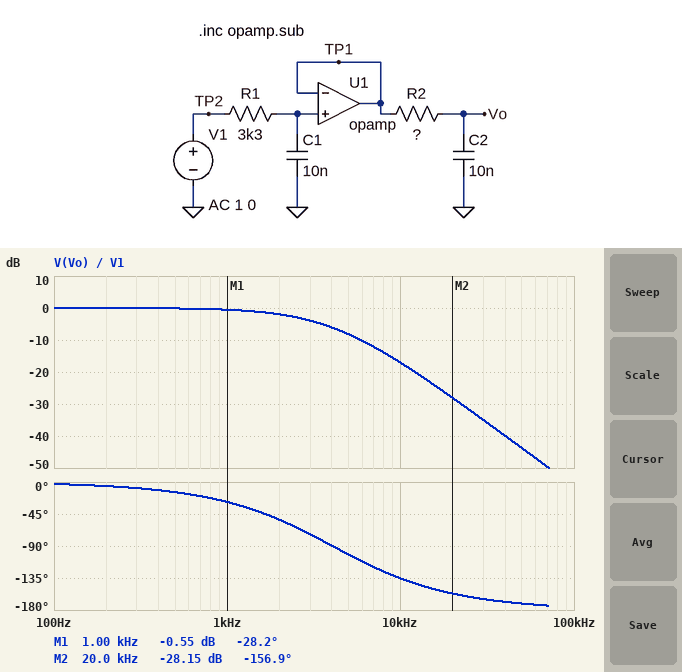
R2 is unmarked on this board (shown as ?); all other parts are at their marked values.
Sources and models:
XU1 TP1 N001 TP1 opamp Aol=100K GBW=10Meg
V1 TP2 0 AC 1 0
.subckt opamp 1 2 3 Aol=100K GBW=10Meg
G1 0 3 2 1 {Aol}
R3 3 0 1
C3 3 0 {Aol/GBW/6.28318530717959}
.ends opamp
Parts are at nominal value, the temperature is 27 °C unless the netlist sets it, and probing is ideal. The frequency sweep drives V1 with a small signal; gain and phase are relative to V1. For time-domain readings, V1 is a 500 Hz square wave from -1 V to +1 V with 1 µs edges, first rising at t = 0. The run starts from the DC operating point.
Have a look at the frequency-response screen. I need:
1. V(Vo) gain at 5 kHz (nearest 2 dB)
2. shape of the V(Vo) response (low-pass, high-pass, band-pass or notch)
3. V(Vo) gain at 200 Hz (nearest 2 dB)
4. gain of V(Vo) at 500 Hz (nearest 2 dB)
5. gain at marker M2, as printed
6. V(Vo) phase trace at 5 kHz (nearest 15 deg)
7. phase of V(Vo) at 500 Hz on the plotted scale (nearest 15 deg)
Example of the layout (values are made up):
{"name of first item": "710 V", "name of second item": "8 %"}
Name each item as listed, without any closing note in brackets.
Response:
{"V(Vo) gain at 5 kHz": "-8 dB", "shape of the V(Vo) response": "low-pass", "V(Vo) gain at 200 Hz": "0 dB", "gain of V(Vo) at 500 Hz": "0 dB", "gain at marker M2, as printed": "-28.15 dB", "V(Vo) phase trace at 5 kHz": "-105 deg", "phase of V(Vo) at 500 Hz on the plotted scale": "-15 deg"}
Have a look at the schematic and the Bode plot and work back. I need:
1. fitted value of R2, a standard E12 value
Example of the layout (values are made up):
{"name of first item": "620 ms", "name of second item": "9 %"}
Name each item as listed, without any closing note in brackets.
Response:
{"fitted value of R2, a standard E12 value": "4.7 kΩ"}
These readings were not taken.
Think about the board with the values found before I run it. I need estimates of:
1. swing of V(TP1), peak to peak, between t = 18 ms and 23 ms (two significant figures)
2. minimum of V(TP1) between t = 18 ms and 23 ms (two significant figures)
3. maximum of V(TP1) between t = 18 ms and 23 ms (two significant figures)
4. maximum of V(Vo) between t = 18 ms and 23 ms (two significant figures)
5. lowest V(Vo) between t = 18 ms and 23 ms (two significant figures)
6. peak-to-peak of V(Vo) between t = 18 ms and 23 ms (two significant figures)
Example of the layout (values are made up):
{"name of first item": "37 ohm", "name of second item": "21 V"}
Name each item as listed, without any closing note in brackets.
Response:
{"swing of V(TP1), peak to peak, between t = 18 ms and 23 ms": "2.0 V", "minimum of V(TP1) between t = 18 ms and 23 ms": "-1.0 V", "maximum of V(TP1) between t = 18 ms and 23 ms": "1.0 V", "maximum of V(Vo) between t = 18 ms and 23 ms": "1.0 V", "lowest V(Vo) between t = 18 ms and 23 ms": "-1.0 V", "peak-to-peak of V(Vo) between t = 18 ms and 23 ms": "2.0 V"}
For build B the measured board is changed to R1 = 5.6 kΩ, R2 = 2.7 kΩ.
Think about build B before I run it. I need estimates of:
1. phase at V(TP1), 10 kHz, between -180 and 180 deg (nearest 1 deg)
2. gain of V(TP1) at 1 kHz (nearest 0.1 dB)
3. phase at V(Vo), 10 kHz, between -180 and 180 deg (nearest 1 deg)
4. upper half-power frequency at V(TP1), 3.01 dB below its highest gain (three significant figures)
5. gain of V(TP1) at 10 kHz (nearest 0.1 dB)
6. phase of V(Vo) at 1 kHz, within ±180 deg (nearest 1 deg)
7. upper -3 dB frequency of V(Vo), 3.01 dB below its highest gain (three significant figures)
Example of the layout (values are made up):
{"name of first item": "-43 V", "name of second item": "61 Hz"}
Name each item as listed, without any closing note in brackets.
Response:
{"phase at V(TP1), 10 kHz, between -180 and 180 deg": "-74 deg", "gain of V(TP1) at 1 kHz": "-0.5 dB", "phase at V(Vo), 10 kHz, between -180 and 180 deg": "-134 deg", "upper half-power frequency at V(TP1), 3.01 dB below its highest gain": "2.84 kHz", "gain of V(TP1) at 10 kHz": "-11.3 dB", "phase of V(Vo) at 1 kHz, within ±180 deg": "-29 deg", "upper -3 dB frequency of V(Vo), 3.01 dB below its highest gain": "2.40 kHz"}
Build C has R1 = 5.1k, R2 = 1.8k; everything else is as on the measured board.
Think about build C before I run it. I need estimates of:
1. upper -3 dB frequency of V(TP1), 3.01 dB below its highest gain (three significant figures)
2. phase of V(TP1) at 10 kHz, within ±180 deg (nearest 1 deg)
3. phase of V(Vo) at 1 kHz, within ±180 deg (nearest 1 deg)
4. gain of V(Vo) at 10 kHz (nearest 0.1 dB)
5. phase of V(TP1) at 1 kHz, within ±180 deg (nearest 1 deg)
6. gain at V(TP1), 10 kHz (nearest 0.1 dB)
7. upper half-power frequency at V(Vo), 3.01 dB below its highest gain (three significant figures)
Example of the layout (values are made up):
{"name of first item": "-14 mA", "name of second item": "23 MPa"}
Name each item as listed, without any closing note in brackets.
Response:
{"upper -3 dB frequency of V(TP1), 3.01 dB below its highest gain": "3.12 kHz", "phase of V(TP1) at 10 kHz, within ±180 deg": "-73 deg", "phase of V(Vo) at 1 kHz, within ±180 deg": "-24 deg", "gain of V(Vo) at 10 kHz": "-14.1 dB", "phase of V(TP1) at 1 kHz, within ±180 deg": "-18 deg", "gain at V(TP1), 10 kHz": "-10.5 dB", "upper half-power frequency at V(Vo), 3.01 dB below its highest gain": "2.82 kHz"}
